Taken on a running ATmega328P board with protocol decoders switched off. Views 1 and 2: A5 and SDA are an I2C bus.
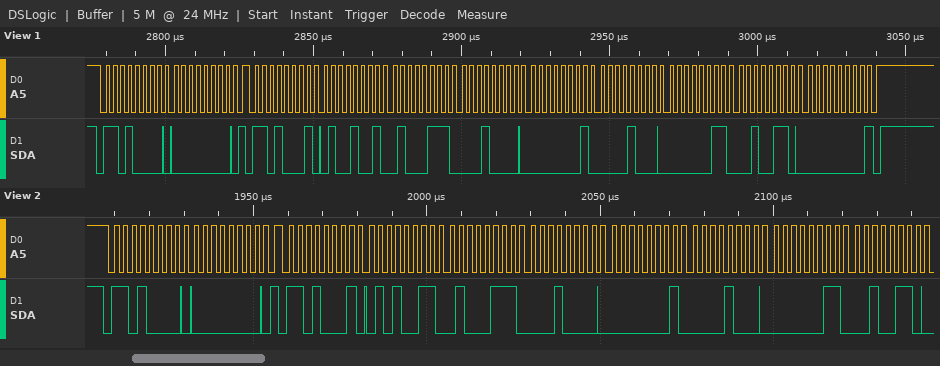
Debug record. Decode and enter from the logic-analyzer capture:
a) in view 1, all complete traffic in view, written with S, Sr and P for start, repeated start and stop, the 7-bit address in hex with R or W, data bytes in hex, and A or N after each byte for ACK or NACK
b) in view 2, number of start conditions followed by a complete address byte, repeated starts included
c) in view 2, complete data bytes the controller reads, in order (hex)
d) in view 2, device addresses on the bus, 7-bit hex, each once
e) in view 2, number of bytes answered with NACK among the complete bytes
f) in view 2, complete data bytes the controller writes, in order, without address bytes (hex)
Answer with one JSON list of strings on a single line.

["S 68W A 00 A Sr 68R A 49 A 47 A 10 A 01 A 08 A 03 A 26 A 00 N P", "2", "53 47 10 01 08 03 26", "0x68", "0", "00"]
